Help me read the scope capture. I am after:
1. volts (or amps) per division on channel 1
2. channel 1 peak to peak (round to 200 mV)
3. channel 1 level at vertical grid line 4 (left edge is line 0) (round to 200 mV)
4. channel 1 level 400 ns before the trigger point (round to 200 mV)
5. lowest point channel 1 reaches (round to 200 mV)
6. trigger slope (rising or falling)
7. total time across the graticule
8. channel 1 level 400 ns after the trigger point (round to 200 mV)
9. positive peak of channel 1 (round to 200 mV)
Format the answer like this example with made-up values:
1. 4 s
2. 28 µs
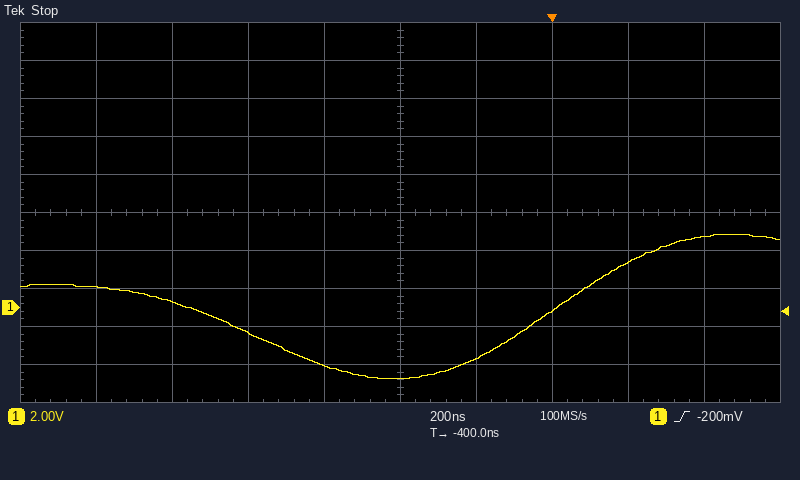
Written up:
1. 2 V
2. 7.6 V
3. -3.0 V
4. -3.8 V
5. -3.8 V
6. rising
7. 2 µs
8. 3.8 V
9. 3.8 V
